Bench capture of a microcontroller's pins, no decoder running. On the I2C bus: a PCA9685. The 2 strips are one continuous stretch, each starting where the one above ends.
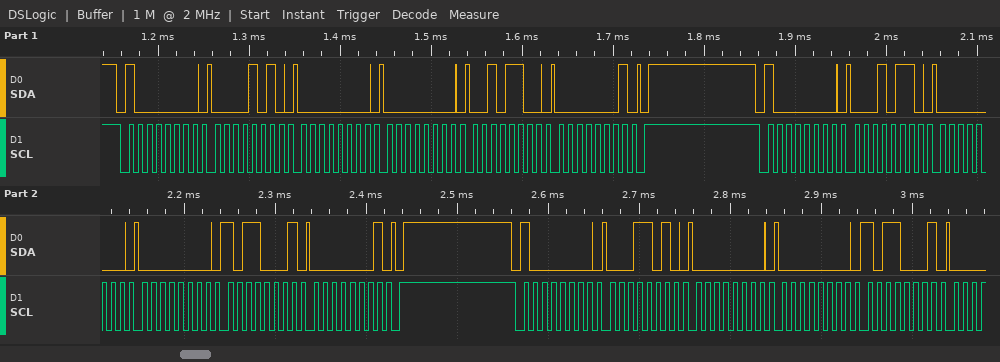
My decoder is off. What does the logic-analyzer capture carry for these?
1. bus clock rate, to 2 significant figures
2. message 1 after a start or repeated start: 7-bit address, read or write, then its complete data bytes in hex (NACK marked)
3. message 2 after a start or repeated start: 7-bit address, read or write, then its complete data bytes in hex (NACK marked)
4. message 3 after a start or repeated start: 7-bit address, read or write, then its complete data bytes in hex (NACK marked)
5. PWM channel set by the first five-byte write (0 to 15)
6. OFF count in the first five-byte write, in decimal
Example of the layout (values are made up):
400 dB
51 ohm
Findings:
100 kHz
0x40 write: 0A 00 00 2C 01
0x40 write: 16 00 00 B1 01
0x40 write: 1A 00 00 B1
1
300
